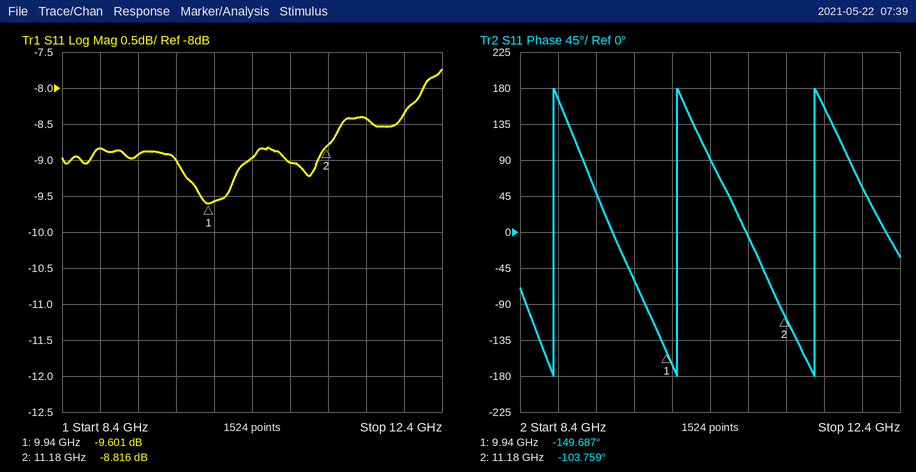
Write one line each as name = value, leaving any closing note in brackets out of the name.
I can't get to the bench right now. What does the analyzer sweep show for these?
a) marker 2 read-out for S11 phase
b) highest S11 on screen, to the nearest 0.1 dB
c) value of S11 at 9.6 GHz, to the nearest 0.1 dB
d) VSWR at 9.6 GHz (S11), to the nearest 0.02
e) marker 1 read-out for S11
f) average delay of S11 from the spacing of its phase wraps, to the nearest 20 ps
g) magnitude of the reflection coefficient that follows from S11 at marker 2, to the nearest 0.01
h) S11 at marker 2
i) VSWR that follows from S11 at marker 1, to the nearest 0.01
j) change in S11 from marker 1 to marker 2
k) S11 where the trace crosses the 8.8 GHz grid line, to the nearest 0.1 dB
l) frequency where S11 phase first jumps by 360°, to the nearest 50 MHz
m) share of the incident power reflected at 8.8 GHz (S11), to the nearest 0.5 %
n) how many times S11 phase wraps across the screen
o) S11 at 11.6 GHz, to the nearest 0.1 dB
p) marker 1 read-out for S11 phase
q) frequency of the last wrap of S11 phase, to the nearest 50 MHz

marker 2 read-out for S11 phase = -103.759°
highest S11 on screen, to the nearest 0.1 dB = -7.7 dB
value of S11 at 9.6 GHz, to the nearest 0.1 dB = -9.0 dB
VSWR at 9.6 GHz (S11), to the nearest 0.02 = 2.10
marker 1 read-out for S11 = -9.601 dB
average delay of S11 from the spacing of its phase wraps, to the nearest 20 ps = 720 ps
magnitude of the reflection coefficient that follows from S11 at marker 2, to the nearest 0.01 = 0.36
S11 at marker 2 = -8.816 dB
VSWR that follows from S11 at marker 1, to the nearest 0.01 = 1.99
change in S11 from marker 1 to marker 2 = 0.785 dB
S11 where the trace crosses the 8.8 GHz grid line, to the nearest 0.1 dB = -8.8 dB
frequency where S11 phase first jumps by 360°, to the nearest 50 MHz = 8.75 GHz
share of the incident power reflected at 8.8 GHz (S11), to the nearest 0.5 % = 13.0 %
how many times S11 phase wraps across the screen = 3
S11 at 11.6 GHz, to the nearest 0.1 dB = -8.4 dB
marker 1 read-out for S11 phase = -149.687°
frequency of the last wrap of S11 phase, to the nearest 50 MHz = 11.50 GHz
